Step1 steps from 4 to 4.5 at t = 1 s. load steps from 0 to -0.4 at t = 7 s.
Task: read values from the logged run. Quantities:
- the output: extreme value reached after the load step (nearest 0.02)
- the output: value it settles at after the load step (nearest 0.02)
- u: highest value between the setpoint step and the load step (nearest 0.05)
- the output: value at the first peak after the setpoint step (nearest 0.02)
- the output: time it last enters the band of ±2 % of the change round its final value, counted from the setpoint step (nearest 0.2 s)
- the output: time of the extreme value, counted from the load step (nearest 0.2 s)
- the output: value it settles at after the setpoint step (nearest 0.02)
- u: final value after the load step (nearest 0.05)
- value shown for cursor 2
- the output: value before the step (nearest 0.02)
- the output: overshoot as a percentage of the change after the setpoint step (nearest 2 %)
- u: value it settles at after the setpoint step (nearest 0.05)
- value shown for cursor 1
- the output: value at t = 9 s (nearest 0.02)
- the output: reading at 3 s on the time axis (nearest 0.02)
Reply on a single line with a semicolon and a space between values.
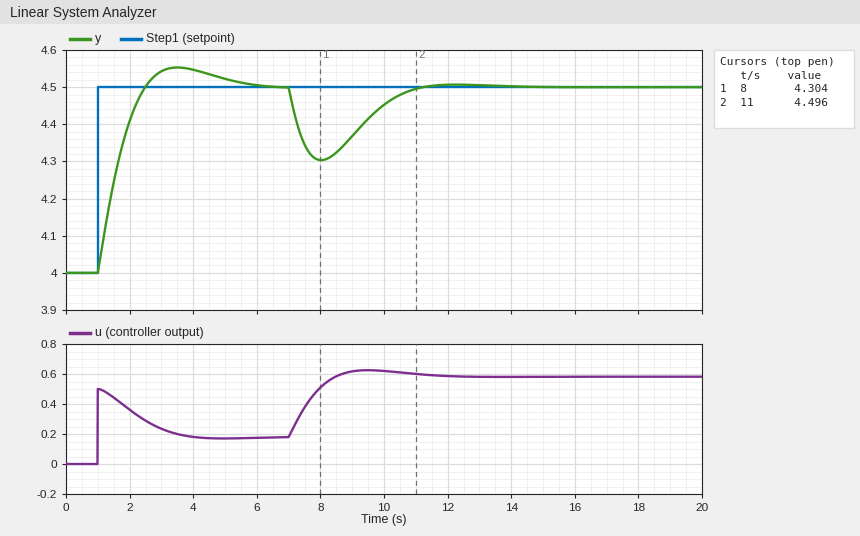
4.30; 4.50; 0.50; 4.56; 4.6 s; 1.0 s; 4.50; 0.60; 4.496; 4.00; 10 %; 0.20; 4.304; 4.36; 4.54
